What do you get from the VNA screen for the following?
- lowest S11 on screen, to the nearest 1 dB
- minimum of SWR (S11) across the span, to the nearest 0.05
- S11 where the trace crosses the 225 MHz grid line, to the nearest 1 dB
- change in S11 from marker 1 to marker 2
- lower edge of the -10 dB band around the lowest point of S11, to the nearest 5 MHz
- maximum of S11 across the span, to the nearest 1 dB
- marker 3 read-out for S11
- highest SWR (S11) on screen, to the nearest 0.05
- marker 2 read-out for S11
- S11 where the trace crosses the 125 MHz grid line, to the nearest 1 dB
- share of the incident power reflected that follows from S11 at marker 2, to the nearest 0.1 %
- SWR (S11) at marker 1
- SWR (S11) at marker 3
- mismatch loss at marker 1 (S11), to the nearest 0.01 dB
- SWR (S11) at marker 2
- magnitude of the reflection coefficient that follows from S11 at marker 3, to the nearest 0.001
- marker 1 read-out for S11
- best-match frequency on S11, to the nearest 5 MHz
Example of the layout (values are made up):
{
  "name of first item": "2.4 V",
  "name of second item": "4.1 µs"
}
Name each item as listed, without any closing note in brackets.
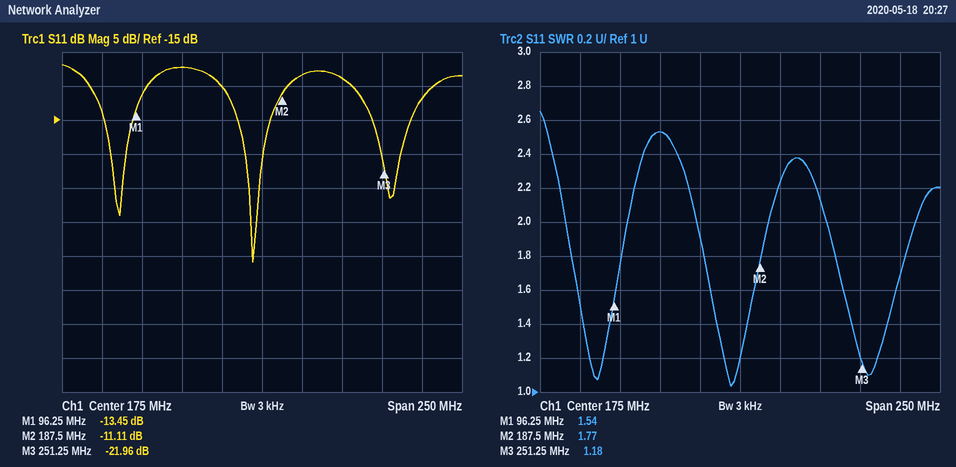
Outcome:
{
  "lowest S11 on screen, to the nearest 1 dB": "-36 dB",
  "minimum of SWR (S11) across the span, to the nearest 0.05": "1.05",
  "S11 where the trace crosses the 225 MHz grid line, to the nearest 1 dB": "-9 dB",
  "change in S11 from marker 1 to marker 2": "2.34 dB",
  "lower edge of the -10 dB band around the lowest point of S11, to the nearest 5 MHz": "150 MHz",
  "maximum of S11 across the span, to the nearest 1 dB": "-7 dB",
  "marker 3 read-out for S11": "-21.96 dB",
  "highest SWR (S11) on screen, to the nearest 0.05": "2.65",
  "marker 2 read-out for S11": "-11.11 dB",
  "S11 where the trace crosses the 125 MHz grid line, to the nearest 1 dB": "-7 dB",
  "share of the incident power reflected that follows from S11 at marker 2, to the nearest 0.1 %": "7.7 %",
  "SWR (S11) at marker 1": "1.54",
  "SWR (S11) at marker 3": "1.18",
  "mismatch loss at marker 1 (S11), to the nearest 0.01 dB": "0.20 dB",
  "SWR (S11) at marker 2": "1.77",
  "magnitude of the reflection coefficient that follows from S11 at marker 3, to the nearest 0.001": "0.080",
  "marker 1 read-out for S11": "-13.45 dB",
  "best-match frequency on S11, to the nearest 5 MHz": "170 MHz"
}
